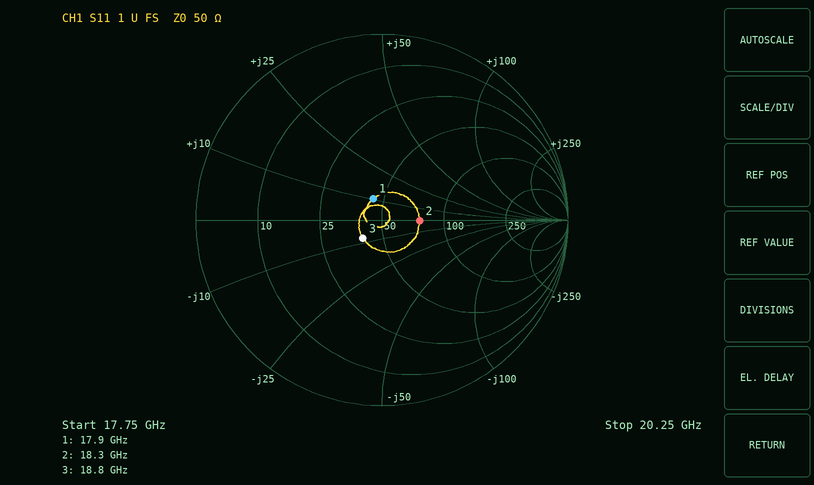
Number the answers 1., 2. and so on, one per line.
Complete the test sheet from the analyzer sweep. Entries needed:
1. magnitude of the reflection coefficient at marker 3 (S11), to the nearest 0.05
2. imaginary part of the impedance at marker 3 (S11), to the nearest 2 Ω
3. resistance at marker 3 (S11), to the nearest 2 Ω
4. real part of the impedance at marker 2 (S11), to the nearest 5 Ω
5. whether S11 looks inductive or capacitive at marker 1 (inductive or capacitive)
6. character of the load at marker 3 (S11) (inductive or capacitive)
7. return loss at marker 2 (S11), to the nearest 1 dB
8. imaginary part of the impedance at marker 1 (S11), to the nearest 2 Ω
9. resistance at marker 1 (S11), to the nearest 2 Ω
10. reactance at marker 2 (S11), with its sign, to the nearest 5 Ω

1. 0.15
2. -8 Ω
3. 40 Ω
4. 75 Ω
5. inductive
6. capacitive
7. 14 dB
8. +10 Ω
9. 44 Ω
10. 0 Ω
